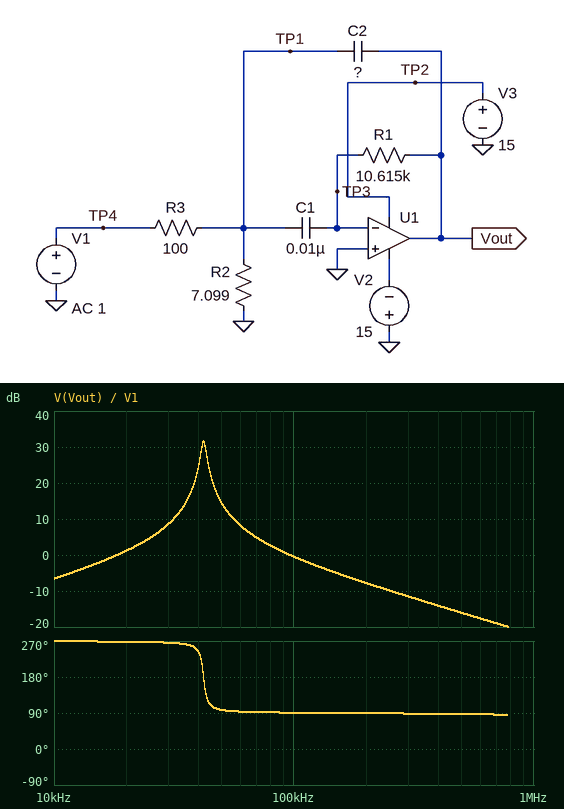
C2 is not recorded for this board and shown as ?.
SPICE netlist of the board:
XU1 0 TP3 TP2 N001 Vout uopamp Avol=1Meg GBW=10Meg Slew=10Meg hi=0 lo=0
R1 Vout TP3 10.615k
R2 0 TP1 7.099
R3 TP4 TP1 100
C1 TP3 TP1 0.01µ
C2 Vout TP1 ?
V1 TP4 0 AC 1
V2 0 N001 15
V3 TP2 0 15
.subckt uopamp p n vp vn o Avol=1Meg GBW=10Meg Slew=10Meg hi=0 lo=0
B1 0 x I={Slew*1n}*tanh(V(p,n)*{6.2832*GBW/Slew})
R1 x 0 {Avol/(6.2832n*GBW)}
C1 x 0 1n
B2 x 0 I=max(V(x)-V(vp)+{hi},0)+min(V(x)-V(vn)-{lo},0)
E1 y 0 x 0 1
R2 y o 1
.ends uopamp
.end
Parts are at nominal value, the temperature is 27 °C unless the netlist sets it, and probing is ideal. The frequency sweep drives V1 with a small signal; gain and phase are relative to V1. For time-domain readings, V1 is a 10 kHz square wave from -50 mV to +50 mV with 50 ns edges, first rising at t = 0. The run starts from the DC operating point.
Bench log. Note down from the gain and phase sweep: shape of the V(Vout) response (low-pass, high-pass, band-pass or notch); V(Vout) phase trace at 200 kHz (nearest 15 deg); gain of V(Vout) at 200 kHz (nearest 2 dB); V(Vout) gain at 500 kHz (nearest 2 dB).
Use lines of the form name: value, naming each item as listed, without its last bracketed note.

shape of the V(Vout) response: band-pass
V(Vout) phase trace at 200 kHz: 90 deg
gain of V(Vout) at 200 kHz: -8 dB
V(Vout) gain at 500 kHz: -16 dB
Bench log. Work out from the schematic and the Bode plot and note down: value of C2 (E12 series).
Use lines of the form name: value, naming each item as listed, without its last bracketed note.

value of C2: 18 nF
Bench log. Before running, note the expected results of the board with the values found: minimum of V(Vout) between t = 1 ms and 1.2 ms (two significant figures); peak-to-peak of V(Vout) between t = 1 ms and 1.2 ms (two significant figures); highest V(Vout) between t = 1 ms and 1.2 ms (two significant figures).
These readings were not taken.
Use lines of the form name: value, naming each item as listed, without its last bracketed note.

minimum of V(Vout) between t = 1 ms and 1.2 ms: -110 mV
peak-to-peak of V(Vout) between t = 1 ms and 1.2 ms: 220 mV
highest V(Vout) between t = 1 ms and 1.2 ms: 110 mV
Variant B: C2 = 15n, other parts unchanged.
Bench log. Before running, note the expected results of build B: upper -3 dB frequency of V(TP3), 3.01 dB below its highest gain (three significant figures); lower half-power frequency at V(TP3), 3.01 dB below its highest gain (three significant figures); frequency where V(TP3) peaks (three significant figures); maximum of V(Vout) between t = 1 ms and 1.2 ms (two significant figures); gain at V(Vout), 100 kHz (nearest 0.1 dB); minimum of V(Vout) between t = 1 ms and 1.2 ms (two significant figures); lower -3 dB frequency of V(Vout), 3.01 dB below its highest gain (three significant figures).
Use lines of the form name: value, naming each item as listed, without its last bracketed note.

upper -3 dB frequency of V(TP3), 3.01 dB below its highest gain: 46.6 kHz
lower half-power frequency at V(TP3), 3.01 dB below its highest gain: 44.5 kHz
frequency where V(TP3) peaks: 45.5 kHz
maximum of V(Vout) between t = 1 ms and 1.2 ms: 170 mV
gain at V(Vout), 100 kHz: 1.2 dB
minimum of V(Vout) between t = 1 ms and 1.2 ms: -170 mV
lower -3 dB frequency of V(Vout), 3.01 dB below its highest gain: 44.4 kHz
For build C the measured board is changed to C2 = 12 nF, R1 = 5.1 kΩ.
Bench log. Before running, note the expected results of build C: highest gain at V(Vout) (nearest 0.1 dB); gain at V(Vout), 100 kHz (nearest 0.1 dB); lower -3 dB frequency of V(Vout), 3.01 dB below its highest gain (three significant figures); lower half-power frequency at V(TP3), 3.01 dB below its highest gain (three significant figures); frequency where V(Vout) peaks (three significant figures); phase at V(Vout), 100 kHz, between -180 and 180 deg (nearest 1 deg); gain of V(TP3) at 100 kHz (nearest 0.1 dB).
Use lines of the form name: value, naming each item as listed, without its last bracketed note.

highest gain at V(Vout): 27.3 dB
gain at V(Vout), 100 kHz: 7.2 dB
lower -3 dB frequency of V(Vout), 3.01 dB below its highest gain: 69.8 kHz
lower half-power frequency at V(TP3), 3.01 dB below its highest gain: 69.9 kHz
frequency where V(Vout) peaks: 72.1 kHz
phase at V(Vout), 100 kHz, between -180 and 180 deg: 95 deg
gain of V(TP3) at 100 kHz: -32.8 dB
